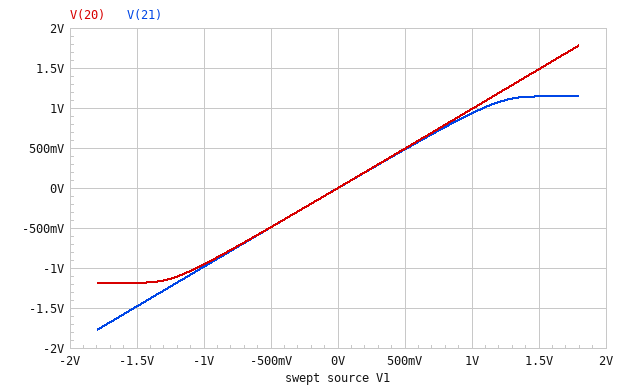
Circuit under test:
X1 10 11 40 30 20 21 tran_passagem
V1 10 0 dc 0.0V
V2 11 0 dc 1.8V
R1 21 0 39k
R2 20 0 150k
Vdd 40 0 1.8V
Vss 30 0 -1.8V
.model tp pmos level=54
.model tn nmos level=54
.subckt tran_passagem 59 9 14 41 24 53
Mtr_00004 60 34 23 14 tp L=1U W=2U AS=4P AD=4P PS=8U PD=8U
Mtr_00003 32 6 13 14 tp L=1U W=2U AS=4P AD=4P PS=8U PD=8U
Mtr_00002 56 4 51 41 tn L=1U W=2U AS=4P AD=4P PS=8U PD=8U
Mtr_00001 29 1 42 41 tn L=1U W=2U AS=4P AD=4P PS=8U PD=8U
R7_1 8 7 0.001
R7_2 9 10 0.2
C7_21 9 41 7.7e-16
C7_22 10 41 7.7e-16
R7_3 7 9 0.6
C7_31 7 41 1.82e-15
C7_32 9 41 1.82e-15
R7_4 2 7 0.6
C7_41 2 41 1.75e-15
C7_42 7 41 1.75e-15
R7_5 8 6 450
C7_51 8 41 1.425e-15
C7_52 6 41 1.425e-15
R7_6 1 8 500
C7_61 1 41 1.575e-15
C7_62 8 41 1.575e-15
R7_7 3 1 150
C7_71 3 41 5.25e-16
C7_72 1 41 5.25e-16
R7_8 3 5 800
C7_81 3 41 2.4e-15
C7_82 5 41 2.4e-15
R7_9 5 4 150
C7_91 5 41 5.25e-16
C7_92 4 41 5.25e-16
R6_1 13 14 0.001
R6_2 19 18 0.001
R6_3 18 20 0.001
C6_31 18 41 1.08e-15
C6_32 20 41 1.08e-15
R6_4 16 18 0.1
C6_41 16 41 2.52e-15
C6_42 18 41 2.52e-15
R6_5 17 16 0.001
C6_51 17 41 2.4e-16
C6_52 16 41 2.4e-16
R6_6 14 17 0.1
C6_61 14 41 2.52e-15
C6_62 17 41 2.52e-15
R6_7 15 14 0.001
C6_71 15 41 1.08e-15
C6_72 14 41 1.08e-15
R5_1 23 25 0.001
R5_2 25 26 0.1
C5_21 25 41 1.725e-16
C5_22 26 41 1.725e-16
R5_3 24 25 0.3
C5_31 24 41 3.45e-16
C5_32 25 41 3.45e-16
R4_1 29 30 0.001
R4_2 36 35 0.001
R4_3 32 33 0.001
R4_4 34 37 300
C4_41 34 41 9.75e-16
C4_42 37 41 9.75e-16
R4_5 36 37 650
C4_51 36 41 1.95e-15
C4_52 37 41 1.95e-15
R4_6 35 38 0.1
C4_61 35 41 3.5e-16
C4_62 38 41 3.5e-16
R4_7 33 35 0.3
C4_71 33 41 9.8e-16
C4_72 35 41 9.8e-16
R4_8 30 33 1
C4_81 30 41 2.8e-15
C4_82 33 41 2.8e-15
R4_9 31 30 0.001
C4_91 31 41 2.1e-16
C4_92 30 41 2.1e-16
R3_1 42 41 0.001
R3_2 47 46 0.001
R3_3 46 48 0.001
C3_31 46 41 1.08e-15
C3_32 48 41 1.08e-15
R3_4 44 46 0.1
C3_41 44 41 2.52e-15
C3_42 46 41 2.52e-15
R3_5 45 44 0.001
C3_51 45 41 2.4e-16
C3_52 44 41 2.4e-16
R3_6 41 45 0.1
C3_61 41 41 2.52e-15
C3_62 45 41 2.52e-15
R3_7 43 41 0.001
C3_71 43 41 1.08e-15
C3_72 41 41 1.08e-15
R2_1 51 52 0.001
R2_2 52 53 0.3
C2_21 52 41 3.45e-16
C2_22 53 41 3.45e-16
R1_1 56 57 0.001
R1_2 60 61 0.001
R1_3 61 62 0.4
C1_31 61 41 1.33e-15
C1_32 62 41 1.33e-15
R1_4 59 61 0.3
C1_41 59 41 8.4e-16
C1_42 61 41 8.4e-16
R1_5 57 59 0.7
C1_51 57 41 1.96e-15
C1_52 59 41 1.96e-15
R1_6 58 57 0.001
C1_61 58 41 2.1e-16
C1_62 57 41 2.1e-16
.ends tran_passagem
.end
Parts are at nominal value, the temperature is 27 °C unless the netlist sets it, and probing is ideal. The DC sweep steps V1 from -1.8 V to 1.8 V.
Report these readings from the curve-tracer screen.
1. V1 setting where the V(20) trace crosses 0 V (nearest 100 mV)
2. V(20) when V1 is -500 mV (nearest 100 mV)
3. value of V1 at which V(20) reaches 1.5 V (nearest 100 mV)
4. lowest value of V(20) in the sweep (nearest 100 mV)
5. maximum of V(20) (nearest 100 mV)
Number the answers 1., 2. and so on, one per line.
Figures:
1. 0 V
2. -500 mV
3. 1.5 V
4. -1.2 V
5. 1.8 V
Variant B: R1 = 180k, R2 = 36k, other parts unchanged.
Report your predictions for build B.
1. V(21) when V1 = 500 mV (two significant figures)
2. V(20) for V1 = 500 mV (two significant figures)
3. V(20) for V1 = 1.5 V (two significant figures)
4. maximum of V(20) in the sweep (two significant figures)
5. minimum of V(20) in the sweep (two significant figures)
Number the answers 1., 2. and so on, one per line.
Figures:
1. 500 mV
2. 470 mV
3. 1.4 V
4. 1.7 V
5. -1.0 V
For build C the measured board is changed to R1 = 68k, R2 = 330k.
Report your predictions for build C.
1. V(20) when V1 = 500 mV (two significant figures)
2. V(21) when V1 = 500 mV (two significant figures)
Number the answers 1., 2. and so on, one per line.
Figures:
1. 500 mV
2. 490 mV
